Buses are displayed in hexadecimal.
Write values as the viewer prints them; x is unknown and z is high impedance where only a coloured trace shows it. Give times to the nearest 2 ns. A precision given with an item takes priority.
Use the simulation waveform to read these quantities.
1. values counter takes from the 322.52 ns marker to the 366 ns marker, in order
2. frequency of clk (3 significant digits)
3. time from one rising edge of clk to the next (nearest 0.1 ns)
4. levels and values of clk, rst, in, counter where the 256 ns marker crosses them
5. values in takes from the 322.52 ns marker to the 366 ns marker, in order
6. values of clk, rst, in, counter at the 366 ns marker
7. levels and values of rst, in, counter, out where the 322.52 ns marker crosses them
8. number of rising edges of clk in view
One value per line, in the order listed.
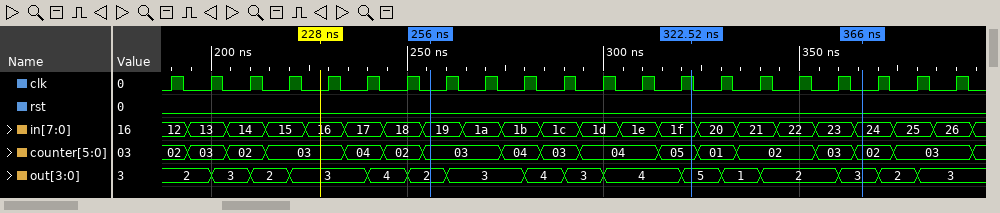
05, 01, 02, 03, 02
100 MHz
10 ns
clk=0, rst=0, in=19, counter=03
1f, 20, 21, 22, 23, 24
clk=0, rst=0, in=24, counter=02
rst=0, in=1f, counter=05, out=5
21
